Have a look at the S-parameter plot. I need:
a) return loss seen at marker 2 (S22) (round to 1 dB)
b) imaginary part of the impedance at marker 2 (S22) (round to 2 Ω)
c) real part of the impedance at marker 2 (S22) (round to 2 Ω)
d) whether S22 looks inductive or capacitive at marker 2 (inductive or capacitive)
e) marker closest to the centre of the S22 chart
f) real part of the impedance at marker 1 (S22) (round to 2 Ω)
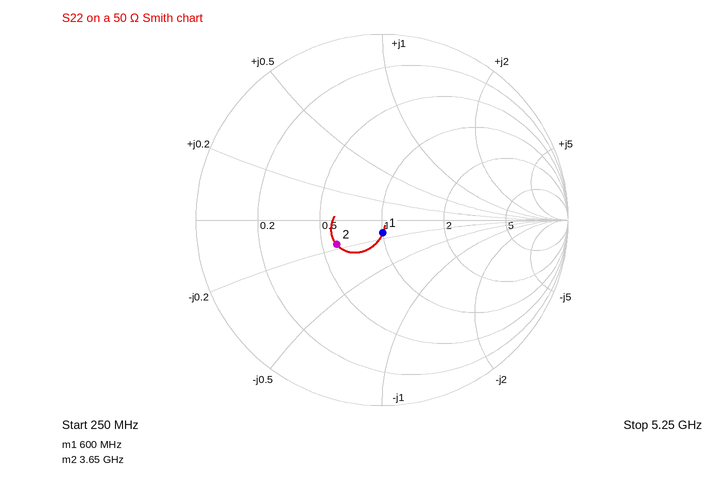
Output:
11 dB
-8 Ω
30 Ω
capacitive
marker 1
50 Ω
